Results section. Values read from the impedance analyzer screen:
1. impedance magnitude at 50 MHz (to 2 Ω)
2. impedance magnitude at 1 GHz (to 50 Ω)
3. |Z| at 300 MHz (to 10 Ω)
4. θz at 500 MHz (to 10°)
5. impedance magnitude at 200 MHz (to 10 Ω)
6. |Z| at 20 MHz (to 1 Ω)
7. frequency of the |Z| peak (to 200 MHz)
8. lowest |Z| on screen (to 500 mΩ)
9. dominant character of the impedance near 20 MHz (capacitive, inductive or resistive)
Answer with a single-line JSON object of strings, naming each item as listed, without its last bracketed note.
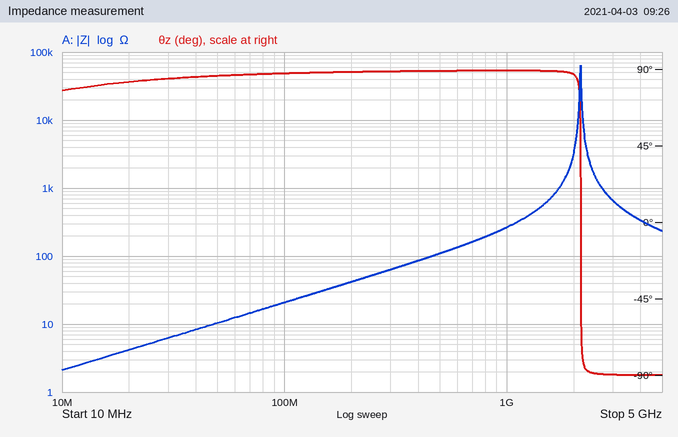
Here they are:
{"impedance magnitude at 50 MHz": "10 Ω", "impedance magnitude at 1 GHz": "250 Ω", "|Z| at 300 MHz": "60 Ω", "θz at 500 MHz": "90°", "impedance magnitude at 200 MHz": "40 Ω", "|Z| at 20 MHz": "4 Ω", "frequency of the |Z| peak": "2.2 GHz", "lowest |Z| on screen": "2.0 Ω", "dominant character of the impedance near 20 MHz": "inductive"}
